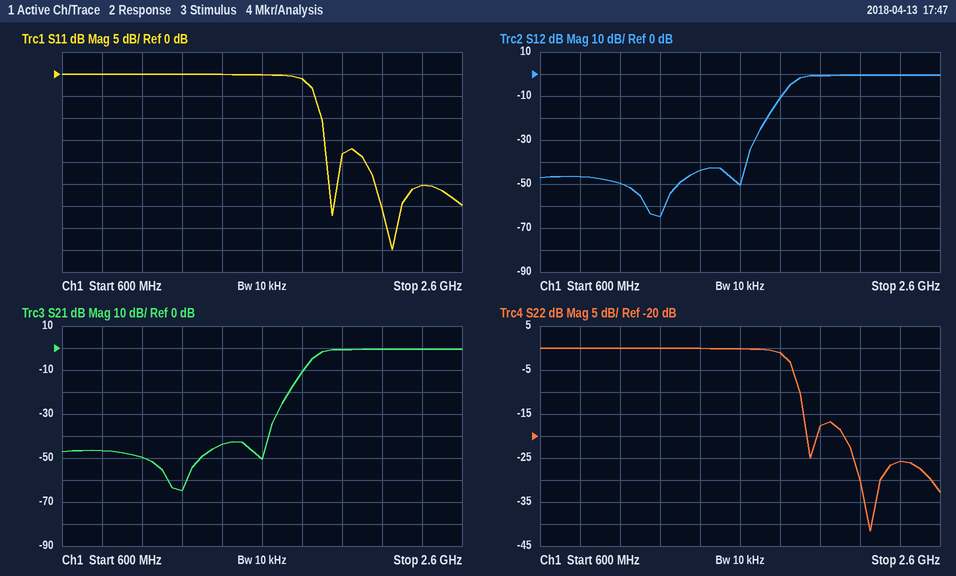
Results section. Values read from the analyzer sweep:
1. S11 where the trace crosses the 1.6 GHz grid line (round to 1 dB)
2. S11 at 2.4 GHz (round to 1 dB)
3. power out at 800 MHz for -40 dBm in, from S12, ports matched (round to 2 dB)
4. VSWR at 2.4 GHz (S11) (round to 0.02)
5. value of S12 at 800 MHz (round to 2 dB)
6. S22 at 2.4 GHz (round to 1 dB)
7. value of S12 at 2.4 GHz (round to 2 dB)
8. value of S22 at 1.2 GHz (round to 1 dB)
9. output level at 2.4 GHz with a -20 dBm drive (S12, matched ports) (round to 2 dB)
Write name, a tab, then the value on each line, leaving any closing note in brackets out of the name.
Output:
S11 where the trace crosses the 1.6 GHz grid line	0 dB
S11 at 2.4 GHz	-25 dB
power out at 800 MHz for -40 dBm in, from S12, ports matched	-86 dBm
VSWR at 2.4 GHz (S11)	1.12
value of S12 at 800 MHz	-46 dB
S22 at 2.4 GHz	-26 dB
value of S12 at 2.4 GHz	0 dB
value of S22 at 1.2 GHz	0 dB
output level at 2.4 GHz with a -20 dBm drive (S12, matched ports)	-20 dBm
